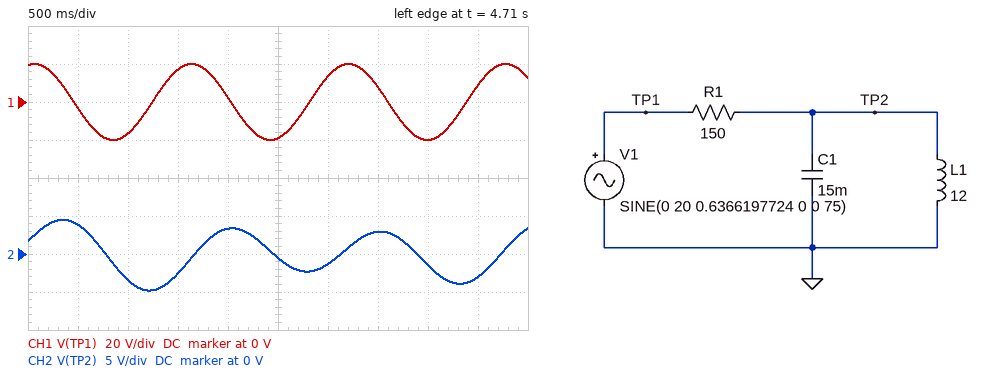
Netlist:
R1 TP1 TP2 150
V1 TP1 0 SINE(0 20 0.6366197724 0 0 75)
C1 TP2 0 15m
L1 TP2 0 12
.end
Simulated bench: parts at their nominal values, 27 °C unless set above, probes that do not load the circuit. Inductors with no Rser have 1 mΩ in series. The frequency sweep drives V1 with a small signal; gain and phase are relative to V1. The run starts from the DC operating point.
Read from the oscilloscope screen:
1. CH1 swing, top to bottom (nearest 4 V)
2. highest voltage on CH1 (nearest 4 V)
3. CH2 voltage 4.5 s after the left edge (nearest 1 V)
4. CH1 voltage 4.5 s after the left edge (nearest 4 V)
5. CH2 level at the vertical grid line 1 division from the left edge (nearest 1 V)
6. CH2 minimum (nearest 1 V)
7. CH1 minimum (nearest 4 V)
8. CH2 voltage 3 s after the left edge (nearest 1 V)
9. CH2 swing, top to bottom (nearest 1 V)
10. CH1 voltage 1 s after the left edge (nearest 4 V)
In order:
40 V
20 V
-3 V
8 V
4 V
-5 V
-20 V
-1 V
9 V
-16 V
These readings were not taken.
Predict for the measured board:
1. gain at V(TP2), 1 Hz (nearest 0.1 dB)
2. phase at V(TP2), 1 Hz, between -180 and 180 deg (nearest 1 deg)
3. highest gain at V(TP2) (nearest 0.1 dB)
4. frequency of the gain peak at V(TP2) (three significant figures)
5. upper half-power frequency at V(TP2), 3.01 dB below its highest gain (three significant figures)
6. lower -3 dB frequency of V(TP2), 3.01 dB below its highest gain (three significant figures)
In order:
-21.7 dB
-85 deg
0 dB
375 mHz
412 mHz
341 mHz
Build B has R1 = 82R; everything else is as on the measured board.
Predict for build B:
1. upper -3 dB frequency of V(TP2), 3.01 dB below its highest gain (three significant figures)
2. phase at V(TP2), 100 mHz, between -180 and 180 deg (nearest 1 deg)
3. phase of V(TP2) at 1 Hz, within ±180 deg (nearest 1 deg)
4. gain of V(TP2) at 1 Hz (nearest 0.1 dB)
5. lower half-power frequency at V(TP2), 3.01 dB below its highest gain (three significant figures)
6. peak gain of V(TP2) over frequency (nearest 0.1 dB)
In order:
445 mHz
84 deg
-81 deg
-16.5 dB
316 mHz
0 dB
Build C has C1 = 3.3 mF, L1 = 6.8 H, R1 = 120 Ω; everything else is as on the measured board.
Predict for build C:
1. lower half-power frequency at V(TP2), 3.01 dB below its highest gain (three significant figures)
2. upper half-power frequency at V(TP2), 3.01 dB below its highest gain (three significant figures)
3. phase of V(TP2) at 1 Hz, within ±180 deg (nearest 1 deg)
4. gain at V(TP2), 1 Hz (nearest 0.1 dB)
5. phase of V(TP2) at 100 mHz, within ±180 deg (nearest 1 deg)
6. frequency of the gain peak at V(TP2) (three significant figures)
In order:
880 mHz
1.28 Hz
18 deg
-0.4 dB
88 deg
1.06 Hz
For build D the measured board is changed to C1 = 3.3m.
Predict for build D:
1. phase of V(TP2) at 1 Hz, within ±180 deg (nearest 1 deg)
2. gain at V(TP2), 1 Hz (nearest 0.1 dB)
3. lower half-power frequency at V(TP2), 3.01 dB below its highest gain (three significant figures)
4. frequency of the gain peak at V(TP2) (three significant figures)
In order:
-48 deg
-3.5 dB
655 mHz
800 mHz
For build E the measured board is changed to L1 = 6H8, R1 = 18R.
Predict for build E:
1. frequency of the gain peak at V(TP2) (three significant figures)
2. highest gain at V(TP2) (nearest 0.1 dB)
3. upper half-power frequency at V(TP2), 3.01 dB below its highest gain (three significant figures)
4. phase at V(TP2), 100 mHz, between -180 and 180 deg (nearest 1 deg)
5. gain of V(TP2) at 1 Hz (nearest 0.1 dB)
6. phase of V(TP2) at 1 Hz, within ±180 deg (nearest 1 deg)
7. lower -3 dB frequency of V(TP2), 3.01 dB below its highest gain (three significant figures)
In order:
498 mHz
0 dB
874 mHz
76 deg
-4.2 dB
-52 deg
284 mHz
